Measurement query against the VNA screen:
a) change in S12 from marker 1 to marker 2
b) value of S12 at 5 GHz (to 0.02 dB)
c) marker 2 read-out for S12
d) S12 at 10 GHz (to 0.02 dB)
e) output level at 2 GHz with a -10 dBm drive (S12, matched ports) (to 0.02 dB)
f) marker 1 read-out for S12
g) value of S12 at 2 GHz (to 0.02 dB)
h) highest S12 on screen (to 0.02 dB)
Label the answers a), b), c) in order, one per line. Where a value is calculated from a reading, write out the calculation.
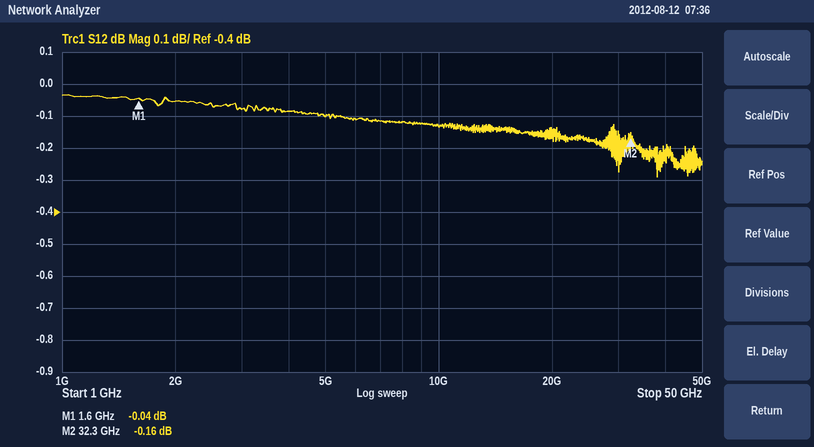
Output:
a) -0.16 − (-0.04) = -0.12 dB
b) -0.10 dB
c) -0.16 dB
d) -0.14 dB
e) -10 dBm + (-0.06 dB) = -10.06 dBm
f) -0.04 dB
g) -0.06 dB
h) -0.04 dB
